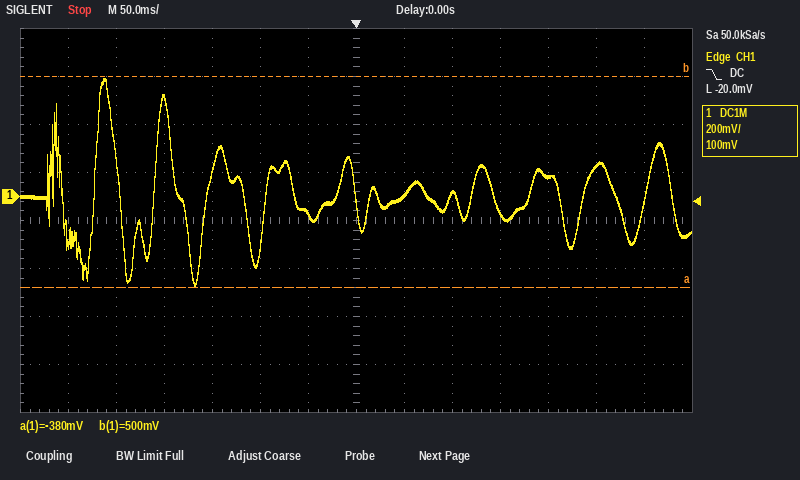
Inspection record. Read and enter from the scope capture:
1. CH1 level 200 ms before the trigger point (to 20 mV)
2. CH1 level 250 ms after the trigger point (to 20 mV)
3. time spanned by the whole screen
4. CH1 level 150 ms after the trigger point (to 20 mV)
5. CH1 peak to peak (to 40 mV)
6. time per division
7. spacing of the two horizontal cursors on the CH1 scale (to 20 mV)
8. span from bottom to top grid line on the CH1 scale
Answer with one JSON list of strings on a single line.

["400 mV", "120 mV", "700 ms", "-60 mV", "880 mV", "50 ms", "880 mV", "1.6 V"]
